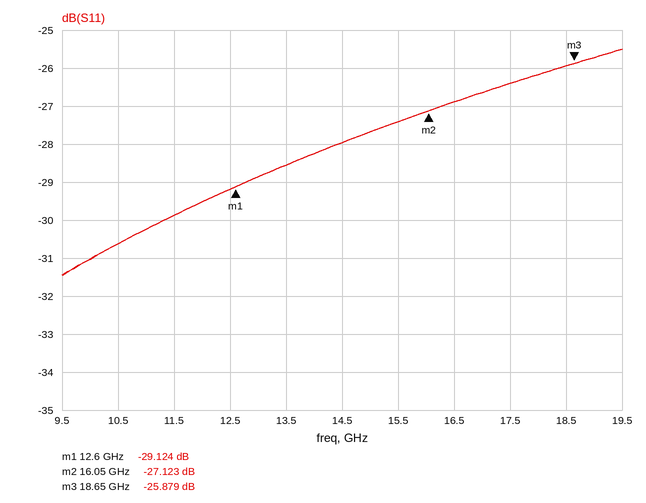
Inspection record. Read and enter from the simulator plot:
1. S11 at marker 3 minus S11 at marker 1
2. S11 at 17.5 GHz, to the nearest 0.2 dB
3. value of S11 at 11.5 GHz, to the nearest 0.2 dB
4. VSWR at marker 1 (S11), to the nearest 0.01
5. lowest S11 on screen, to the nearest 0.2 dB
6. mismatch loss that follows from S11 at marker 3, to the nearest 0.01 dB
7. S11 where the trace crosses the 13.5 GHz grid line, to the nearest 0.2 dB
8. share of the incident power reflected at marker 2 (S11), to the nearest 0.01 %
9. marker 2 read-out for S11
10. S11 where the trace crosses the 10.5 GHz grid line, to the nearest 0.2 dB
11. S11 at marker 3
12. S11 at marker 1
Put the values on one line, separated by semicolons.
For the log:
3.245 dB; -26.4 dB; -29.8 dB; 1.07; -31.4 dB; 0.01 dB; -28.6 dB; 0.19 %; -27.123 dB; -30.6 dB; -25.879 dB; -29.124 dB
